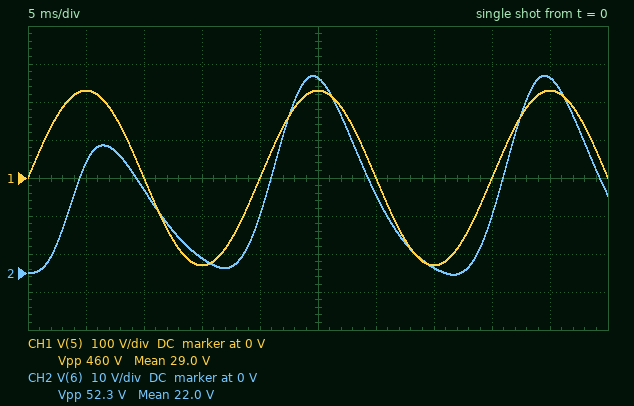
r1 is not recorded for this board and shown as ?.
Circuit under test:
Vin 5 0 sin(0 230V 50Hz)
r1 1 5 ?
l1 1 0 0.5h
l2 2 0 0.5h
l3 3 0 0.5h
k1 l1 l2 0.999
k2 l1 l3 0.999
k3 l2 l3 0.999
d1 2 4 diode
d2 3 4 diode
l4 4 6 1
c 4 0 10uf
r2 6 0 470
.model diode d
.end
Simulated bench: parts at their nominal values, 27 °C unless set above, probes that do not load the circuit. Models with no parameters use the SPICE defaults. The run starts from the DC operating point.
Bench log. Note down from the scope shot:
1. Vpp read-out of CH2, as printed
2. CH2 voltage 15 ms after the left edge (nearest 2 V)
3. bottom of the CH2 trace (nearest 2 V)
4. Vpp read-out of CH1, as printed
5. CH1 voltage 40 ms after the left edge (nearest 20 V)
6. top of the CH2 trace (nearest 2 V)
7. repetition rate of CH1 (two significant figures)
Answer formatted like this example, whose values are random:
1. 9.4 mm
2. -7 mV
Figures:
1. 52.3 V
2. 4 V
3. 0 V
4. 460 V
5. 0 V
6. 52 V
7. 50 Hz
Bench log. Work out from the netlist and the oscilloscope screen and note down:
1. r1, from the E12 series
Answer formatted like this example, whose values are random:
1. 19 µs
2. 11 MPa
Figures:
1. 680 Ω
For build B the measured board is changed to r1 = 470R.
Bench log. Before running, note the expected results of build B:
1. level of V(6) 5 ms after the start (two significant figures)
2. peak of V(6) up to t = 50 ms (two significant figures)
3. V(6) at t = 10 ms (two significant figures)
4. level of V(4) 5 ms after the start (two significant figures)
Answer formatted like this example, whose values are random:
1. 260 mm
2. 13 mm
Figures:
1. 39 V
2. 70 V
3. 29 V
4. 57 V
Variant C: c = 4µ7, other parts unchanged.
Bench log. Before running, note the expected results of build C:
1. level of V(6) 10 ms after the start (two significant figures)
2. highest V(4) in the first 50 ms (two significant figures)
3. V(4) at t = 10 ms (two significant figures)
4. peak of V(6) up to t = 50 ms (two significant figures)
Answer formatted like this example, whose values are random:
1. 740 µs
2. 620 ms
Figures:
1. 1.7 V
2. 55 V
3. -9.3 V
4. 45 V
